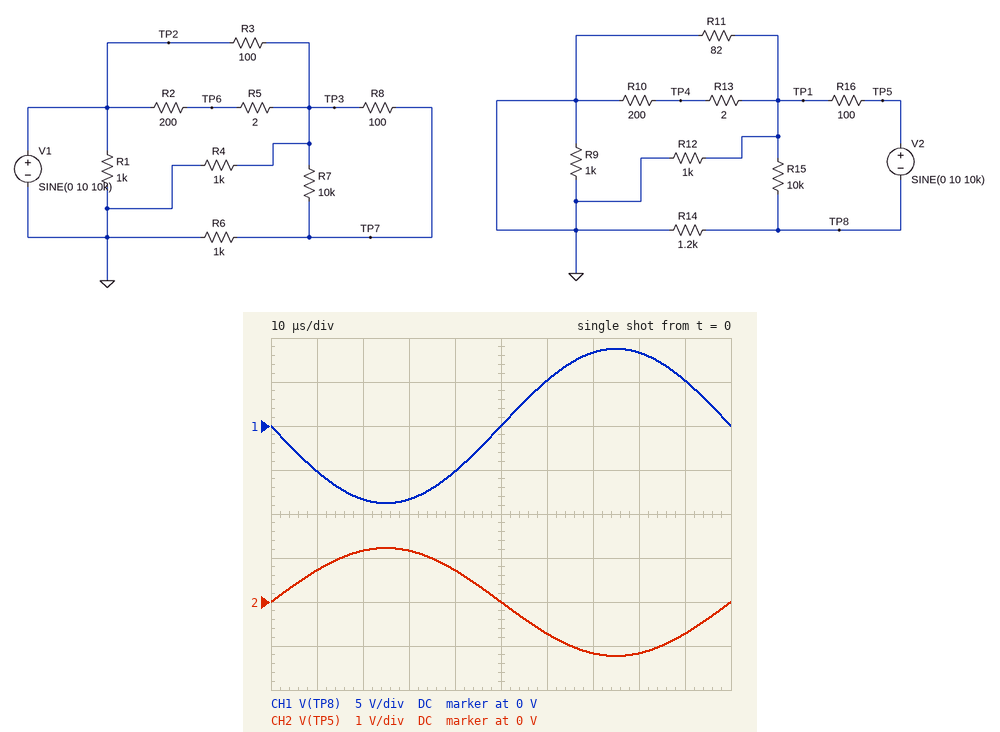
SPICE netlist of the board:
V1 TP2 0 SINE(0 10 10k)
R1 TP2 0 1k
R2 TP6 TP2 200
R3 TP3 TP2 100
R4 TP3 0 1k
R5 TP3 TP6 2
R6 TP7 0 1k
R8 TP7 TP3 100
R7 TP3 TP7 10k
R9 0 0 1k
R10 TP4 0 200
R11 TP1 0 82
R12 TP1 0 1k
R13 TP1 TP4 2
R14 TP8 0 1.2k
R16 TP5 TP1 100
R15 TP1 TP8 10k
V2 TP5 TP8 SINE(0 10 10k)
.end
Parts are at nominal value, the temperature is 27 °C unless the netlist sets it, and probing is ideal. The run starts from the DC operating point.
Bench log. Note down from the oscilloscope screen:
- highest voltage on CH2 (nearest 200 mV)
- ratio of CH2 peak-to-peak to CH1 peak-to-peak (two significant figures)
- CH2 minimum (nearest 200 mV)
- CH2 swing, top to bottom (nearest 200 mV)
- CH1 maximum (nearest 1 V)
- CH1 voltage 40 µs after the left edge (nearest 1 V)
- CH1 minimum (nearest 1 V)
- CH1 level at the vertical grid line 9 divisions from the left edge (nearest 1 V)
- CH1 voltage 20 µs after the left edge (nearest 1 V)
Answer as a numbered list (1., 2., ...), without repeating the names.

1. 1.2 V
2. 0.14
3. -1.2 V
4. 2.4 V
5. 9 V
6. -5 V
7. -9 V
8. 5 V
9. -8 V
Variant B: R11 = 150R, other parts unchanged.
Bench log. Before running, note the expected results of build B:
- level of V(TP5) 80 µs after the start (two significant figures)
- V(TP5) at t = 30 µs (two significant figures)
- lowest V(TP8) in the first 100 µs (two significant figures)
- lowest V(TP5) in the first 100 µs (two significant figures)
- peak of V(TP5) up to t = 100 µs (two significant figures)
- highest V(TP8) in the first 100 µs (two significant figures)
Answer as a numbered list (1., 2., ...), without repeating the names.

1. -1.3 V
2. 1.3 V
3. -8.6 V
4. -1.4 V
5. 1.4 V
6. 8.6 V
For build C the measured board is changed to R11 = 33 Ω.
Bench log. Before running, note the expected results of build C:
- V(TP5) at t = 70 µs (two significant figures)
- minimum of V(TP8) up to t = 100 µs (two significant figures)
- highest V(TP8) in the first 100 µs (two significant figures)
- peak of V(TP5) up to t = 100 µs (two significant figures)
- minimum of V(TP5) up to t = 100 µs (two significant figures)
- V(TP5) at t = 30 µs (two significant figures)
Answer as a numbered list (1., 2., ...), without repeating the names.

1. -990 mV
2. -9.0 V
3. 9.0 V
4. 1.0 V
5. -1.0 V
6. 990 mV
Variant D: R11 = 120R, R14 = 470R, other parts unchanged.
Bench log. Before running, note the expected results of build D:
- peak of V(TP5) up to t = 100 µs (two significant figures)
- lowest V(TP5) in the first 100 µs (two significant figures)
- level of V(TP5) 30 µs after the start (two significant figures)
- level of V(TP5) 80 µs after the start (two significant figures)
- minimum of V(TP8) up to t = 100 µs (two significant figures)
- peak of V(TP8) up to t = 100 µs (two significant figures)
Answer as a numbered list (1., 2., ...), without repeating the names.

1. 2.7 V
2. -2.7 V
3. 2.6 V
4. -2.6 V
5. -7.3 V
6. 7.3 V
